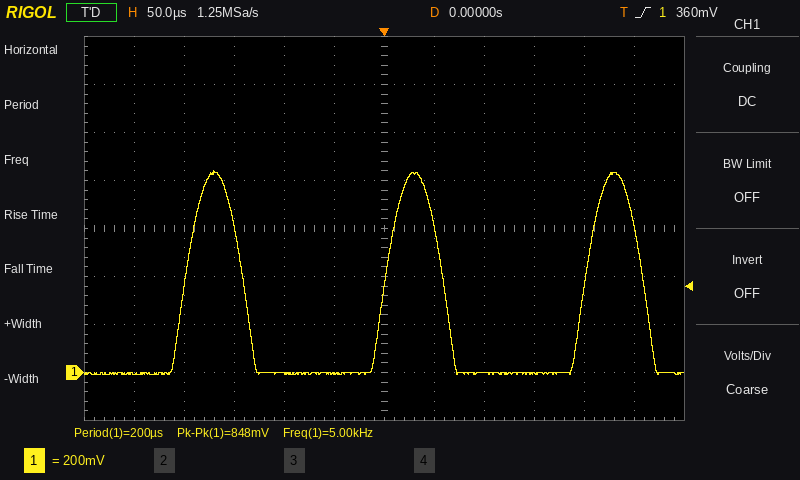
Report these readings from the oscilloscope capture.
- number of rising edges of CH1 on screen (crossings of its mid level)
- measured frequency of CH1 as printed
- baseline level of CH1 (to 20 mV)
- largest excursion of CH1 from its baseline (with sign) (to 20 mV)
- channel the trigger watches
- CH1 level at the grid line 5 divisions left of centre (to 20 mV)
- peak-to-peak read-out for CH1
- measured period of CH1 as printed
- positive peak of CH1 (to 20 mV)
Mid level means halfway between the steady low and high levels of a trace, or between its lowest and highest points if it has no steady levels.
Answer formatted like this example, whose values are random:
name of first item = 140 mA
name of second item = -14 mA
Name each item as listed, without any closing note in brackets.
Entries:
number of rising edges of CH1 on screen = 3
measured frequency of CH1 as printed = 5.00 kHz
baseline level of CH1 = 0 mV
largest excursion of CH1 from its baseline (with sign) = +840 mV
channel the trigger watches = CH1
CH1 level at the grid line 5 divisions left of centre = 0 mV
peak-to-peak read-out for CH1 = 848 mV
measured period of CH1 as printed = 200 µs
positive peak of CH1 = 840 mV
